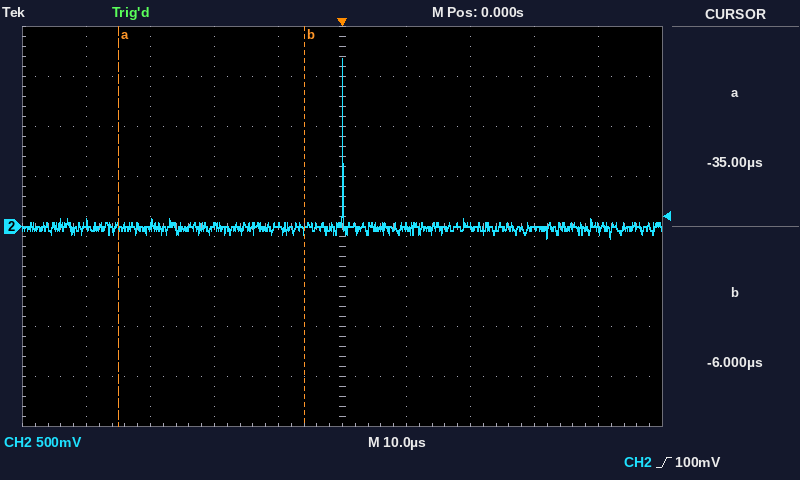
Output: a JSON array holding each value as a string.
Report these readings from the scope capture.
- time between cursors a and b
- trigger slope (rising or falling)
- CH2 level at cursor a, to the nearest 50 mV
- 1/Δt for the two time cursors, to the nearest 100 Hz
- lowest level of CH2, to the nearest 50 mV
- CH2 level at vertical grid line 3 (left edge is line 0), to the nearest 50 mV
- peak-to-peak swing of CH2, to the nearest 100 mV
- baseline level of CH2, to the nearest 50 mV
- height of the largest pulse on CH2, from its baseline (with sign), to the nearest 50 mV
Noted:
["29 µs", "rising", "0 mV", "34.5 kHz", "-100 mV", "0 mV", "1.80 V", "0 mV", "+1.70 V"]
